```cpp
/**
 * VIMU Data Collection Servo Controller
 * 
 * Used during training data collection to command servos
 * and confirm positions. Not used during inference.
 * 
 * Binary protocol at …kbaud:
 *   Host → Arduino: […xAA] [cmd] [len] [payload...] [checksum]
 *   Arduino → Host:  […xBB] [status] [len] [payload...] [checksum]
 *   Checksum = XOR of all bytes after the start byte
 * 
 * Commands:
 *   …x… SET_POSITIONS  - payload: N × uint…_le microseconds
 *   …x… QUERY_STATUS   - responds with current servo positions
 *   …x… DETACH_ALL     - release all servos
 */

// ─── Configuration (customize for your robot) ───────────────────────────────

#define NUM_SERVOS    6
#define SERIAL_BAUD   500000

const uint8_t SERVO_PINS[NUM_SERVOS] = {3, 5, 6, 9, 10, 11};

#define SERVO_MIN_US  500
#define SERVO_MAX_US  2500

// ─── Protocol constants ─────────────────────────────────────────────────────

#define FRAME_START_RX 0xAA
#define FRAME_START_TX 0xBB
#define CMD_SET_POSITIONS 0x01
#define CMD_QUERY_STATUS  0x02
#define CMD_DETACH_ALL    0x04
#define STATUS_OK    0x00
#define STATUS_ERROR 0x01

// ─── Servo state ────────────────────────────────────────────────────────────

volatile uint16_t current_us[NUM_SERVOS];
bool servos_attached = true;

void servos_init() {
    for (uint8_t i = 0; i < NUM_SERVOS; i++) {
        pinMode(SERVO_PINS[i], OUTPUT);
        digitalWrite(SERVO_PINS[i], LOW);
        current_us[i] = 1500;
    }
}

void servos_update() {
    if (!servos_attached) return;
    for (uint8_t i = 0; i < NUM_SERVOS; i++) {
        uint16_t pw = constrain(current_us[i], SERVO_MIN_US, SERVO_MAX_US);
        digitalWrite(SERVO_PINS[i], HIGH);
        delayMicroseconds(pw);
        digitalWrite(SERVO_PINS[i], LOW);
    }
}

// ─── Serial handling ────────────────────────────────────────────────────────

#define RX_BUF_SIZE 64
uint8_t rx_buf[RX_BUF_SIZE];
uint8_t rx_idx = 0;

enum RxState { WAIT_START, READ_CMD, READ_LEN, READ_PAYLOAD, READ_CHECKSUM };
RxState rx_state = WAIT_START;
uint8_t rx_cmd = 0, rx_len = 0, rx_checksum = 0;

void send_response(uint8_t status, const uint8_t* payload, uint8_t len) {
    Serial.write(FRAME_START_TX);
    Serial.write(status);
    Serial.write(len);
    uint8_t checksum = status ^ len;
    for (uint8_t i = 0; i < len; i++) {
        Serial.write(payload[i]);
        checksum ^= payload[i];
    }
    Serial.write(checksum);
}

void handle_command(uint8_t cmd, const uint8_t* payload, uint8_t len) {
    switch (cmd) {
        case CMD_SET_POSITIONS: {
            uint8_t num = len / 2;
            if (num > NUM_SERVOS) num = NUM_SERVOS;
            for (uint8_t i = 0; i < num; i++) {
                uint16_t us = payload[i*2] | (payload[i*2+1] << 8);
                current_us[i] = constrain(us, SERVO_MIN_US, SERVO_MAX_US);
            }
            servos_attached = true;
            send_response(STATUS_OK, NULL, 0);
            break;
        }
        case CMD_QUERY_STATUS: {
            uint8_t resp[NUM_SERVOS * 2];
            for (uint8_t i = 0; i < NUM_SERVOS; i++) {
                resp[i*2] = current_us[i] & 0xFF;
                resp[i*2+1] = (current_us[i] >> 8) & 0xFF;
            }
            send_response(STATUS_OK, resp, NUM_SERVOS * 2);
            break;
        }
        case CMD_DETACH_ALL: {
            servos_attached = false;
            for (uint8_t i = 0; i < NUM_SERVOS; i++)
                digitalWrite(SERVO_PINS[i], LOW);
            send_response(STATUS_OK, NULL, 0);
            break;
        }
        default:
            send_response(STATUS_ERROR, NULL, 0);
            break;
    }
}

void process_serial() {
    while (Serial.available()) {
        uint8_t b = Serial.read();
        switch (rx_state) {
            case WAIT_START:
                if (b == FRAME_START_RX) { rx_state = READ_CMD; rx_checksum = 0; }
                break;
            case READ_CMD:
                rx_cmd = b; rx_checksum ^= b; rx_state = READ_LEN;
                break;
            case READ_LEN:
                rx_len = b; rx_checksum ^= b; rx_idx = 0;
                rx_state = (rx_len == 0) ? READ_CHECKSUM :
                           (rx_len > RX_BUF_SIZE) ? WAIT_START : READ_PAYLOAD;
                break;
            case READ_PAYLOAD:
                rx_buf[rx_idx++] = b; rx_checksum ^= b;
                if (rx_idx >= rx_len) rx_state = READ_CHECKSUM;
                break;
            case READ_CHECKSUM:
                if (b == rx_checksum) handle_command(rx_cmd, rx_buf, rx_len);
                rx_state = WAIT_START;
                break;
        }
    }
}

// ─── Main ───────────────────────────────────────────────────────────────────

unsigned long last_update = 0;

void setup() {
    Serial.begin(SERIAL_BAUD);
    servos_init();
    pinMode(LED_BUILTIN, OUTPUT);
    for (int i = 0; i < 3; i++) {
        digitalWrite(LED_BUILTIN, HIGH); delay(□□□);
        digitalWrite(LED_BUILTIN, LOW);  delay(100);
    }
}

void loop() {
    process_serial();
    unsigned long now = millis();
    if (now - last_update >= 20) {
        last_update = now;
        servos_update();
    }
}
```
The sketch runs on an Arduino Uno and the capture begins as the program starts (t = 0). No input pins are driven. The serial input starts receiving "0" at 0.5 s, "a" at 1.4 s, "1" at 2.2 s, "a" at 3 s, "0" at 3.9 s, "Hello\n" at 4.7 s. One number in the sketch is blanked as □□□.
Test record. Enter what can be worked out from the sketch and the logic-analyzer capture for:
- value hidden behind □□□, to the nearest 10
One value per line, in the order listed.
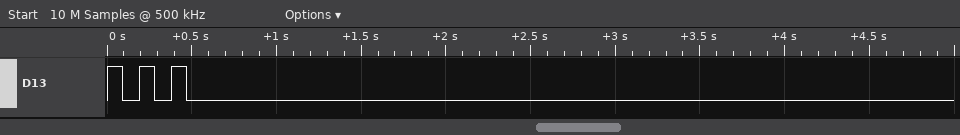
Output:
90
